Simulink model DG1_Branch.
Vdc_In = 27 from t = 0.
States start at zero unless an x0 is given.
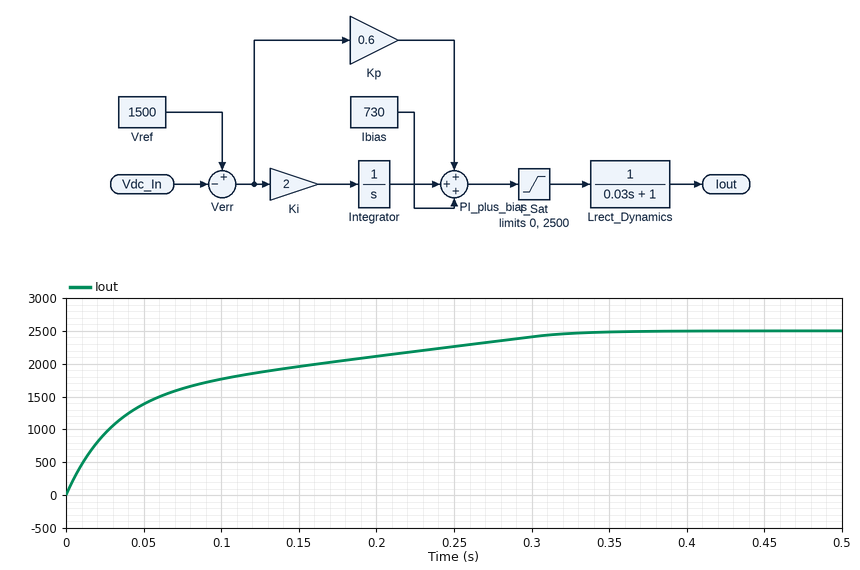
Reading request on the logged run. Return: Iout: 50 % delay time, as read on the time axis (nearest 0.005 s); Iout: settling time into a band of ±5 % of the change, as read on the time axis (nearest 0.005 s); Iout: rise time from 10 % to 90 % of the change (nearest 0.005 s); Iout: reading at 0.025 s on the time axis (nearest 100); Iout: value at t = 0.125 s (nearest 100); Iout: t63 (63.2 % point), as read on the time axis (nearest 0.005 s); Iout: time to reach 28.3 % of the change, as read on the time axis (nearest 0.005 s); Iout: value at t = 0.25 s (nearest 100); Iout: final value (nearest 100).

0.040 s
0.290 s
0.240 s
900
1900
0.070 s
0.015 s
2300
2500
